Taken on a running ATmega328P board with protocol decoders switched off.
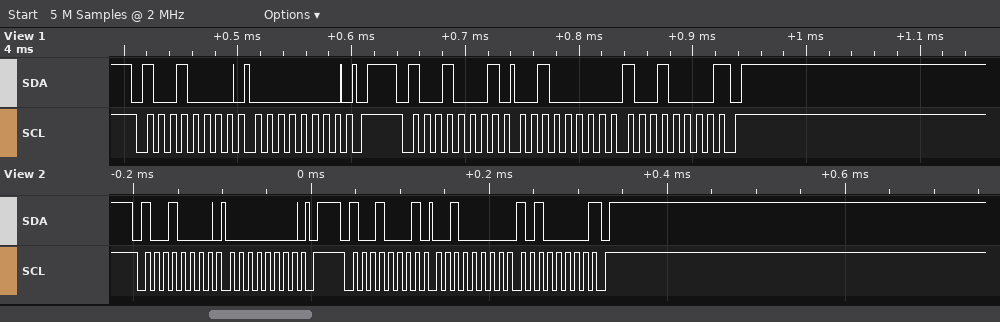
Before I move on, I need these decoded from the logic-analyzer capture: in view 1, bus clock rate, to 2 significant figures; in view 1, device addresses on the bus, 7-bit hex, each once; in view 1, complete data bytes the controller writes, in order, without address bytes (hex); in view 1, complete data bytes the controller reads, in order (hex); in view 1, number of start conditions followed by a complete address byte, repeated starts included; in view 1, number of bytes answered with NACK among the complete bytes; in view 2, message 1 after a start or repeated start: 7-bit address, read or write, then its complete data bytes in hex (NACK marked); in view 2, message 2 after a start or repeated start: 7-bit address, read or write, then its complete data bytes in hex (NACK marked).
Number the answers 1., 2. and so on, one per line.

1. 100 kHz
2. 0x48
3. 00
4. 20 90
5. 2
6. 1
7. 0x48 write: 00
8. 0x48 read: 20 A0 NACK
